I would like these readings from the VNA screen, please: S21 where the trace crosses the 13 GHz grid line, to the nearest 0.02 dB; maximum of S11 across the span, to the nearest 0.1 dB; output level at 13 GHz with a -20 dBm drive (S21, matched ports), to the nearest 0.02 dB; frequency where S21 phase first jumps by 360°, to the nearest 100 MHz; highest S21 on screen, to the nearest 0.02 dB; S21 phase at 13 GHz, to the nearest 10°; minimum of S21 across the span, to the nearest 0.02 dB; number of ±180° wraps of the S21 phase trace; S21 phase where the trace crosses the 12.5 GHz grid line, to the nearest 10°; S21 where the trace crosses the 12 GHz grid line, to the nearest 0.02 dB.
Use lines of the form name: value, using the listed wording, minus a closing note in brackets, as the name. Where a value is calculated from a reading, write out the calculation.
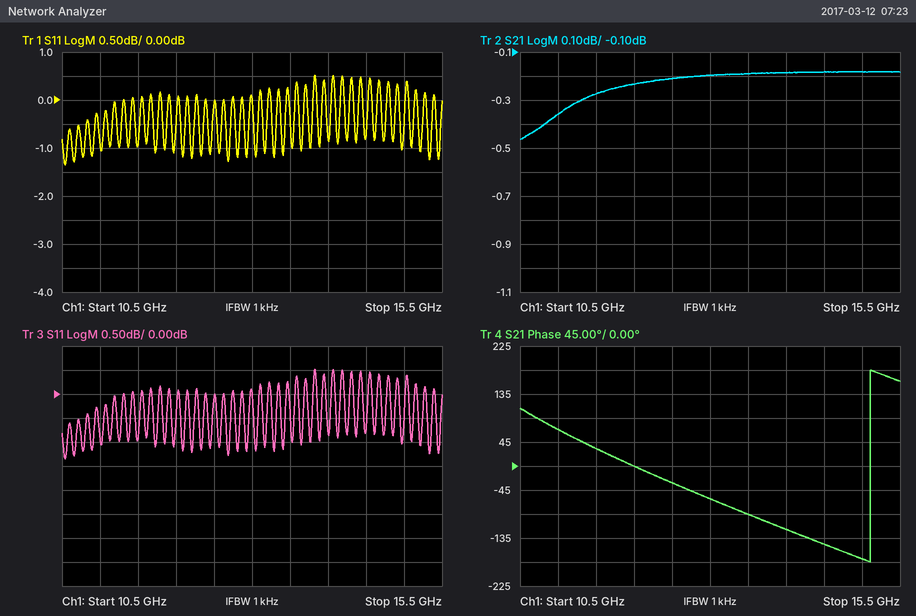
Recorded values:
S21 where the trace crosses the 13 GHz grid line, to the nearest 0.02 dB: -0.20 dB
maximum of S11 across the span, to the nearest 0.1 dB: 0.5 dB
output level at 13 GHz with a -20 dBm drive (S21, matched ports), to the nearest 0.02 dB: -20 dBm + (-0.20 dB) = -20.20 dBm
frequency where S21 phase first jumps by 360°, to the nearest 100 MHz: 15.1 GHz
highest S21 on screen, to the nearest 0.02 dB: -0.18 dB
S21 phase at 13 GHz, to the nearest 10°: -60°
minimum of S21 across the span, to the nearest 0.02 dB: -0.46 dB
number of ±180° wraps of the S21 phase trace: 1
S21 phase where the trace crosses the 12.5 GHz grid line, to the nearest 10°: -30°
S21 where the trace crosses the 12 GHz grid line, to the nearest 0.02 dB: -0.24 dB
